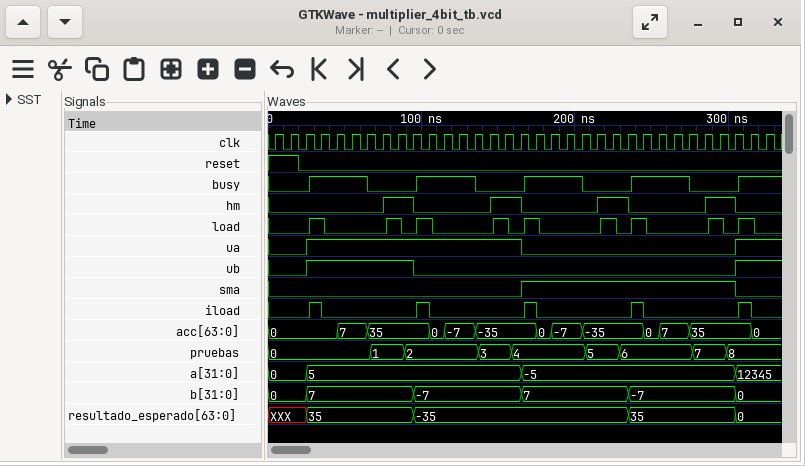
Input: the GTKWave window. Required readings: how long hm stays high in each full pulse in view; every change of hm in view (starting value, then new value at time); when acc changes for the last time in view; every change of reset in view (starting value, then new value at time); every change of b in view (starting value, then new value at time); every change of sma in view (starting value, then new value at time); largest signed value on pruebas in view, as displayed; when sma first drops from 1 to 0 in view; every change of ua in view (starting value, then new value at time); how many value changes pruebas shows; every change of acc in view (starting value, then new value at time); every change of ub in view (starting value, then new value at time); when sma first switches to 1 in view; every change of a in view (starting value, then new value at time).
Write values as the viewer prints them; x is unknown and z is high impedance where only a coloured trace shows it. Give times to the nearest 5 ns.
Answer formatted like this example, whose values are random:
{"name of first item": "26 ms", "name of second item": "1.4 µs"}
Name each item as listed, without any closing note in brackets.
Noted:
{"how long hm stays high in each full pulse in view": "20 ns, 20 ns, 20 ns, 20 ns", "every change of hm in view": "0, 1 at 75 ns, 0 at 95 ns, 1 at 145 ns, 0 at 165 ns, 1 at 215 ns, 0 at 235 ns, 1 at 285 ns, 0 at 305 ns", "when acc changes for the last time in view": "315 ns", "every change of reset in view": "1, 0 at 20 ns", "every change of b in view": "0, 7 at 25 ns, -7 at 95 ns, 7 at 165 ns, -7 at 235 ns, 0 at 305 ns", "every change of sma in view": "0, 1 at 165 ns, 0 at 305 ns", "largest signed value on pruebas in view, as displayed": "8", "when sma first drops from 1 to 0 in view": "305 ns", "every change of ua in view": "0, 1 at 25 ns, 0 at 165 ns, 1 at 305 ns", "how many value changes pruebas shows": "8", "every change of acc in view": "0, 7 at 45 ns, 35 at 65 ns, 0 at 105 ns, -7 at 115 ns, -35 at 135 ns, 0 at 175 ns, -7 at 185 ns, -35 at 205 ns, 0 at 245 ns, 7 at 255 ns, 35 at 275 ns, 0 at 315 ns", "every change of ub in view": "0, 1 at 25 ns, 0 at 95 ns, 1 at 305 ns", "when sma first switches to 1 in view": "165 ns", "every change of a in view": "0, 5 at 25 ns, -5 at 165 ns, 12345 at 305 ns"}
